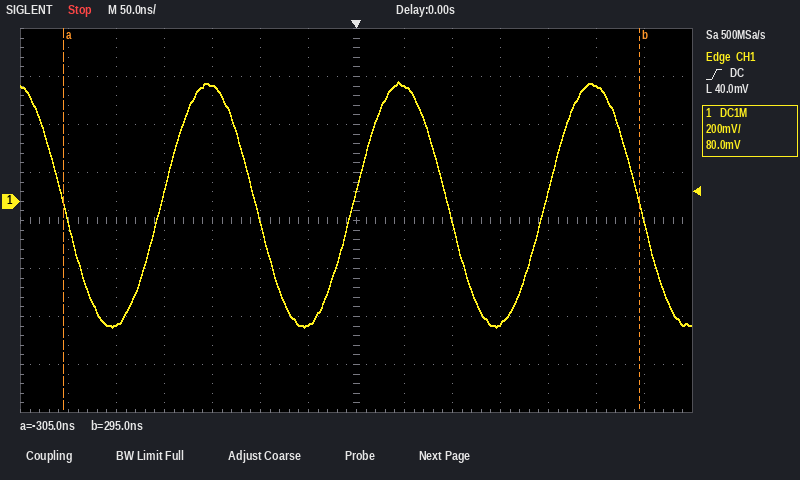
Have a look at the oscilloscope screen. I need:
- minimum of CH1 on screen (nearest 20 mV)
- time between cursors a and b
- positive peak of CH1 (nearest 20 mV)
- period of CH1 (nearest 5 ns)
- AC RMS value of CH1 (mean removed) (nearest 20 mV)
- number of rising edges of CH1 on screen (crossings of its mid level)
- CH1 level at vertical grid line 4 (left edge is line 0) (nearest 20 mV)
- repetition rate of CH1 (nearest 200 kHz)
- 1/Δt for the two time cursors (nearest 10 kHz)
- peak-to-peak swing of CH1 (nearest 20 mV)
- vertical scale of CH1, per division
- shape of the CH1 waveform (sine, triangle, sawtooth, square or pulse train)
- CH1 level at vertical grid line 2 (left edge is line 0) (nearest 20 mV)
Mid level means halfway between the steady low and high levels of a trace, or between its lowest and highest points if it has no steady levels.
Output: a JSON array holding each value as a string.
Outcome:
["-520 mV", "600 ns", "500 mV", "200 ns", "360 mV", "3", "480 mV", "5.0 MHz", "1.67 MHz", "1.02 V", "200 mV", "sine", "-520 mV"]
